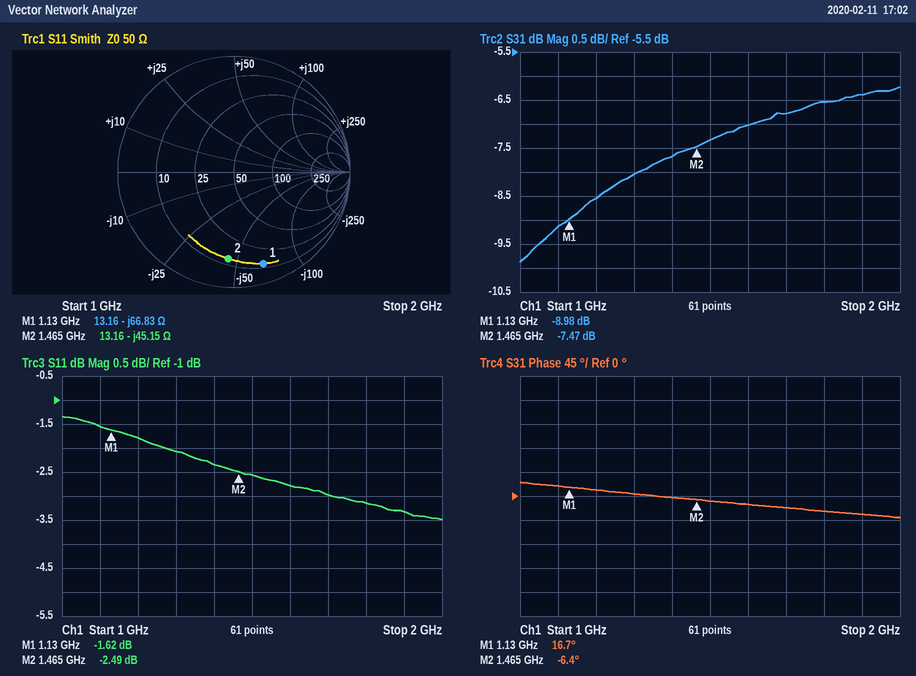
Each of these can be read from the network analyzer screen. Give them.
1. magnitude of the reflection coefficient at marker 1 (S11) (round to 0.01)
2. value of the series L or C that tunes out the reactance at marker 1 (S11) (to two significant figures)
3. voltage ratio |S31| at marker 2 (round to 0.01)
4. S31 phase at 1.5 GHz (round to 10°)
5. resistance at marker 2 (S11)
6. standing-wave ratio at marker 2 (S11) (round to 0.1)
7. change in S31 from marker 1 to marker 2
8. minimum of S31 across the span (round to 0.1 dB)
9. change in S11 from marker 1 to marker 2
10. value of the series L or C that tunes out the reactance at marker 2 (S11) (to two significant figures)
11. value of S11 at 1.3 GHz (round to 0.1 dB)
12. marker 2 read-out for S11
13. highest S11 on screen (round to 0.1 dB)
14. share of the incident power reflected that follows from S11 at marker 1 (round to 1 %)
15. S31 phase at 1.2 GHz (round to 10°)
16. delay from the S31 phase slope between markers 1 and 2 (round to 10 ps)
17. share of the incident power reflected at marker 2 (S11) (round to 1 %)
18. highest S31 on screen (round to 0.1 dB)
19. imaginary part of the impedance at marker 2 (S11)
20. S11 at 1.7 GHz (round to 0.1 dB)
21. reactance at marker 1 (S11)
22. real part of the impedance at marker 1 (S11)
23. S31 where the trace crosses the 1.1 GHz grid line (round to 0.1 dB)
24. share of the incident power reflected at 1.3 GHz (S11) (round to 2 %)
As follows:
0.83
9.4 nH
0.42
-10°
13.16 Ω
7.0
1.51 dB
-9.9 dB
-0.87 dB
4.9 nH
-2.1 dB
-2.49 dB
-1.3 dB
69 %
10°
190 ps
56 %
-6.2 dB
-45.15 Ω
-3.0 dB
-66.83 Ω
13.16 Ω
-9.1 dB
62 %
